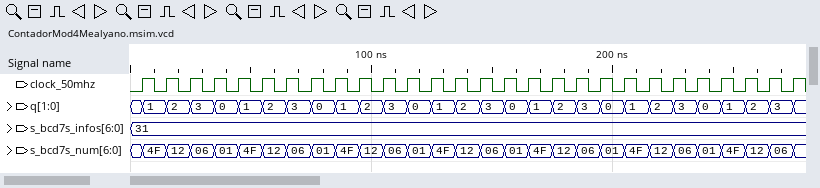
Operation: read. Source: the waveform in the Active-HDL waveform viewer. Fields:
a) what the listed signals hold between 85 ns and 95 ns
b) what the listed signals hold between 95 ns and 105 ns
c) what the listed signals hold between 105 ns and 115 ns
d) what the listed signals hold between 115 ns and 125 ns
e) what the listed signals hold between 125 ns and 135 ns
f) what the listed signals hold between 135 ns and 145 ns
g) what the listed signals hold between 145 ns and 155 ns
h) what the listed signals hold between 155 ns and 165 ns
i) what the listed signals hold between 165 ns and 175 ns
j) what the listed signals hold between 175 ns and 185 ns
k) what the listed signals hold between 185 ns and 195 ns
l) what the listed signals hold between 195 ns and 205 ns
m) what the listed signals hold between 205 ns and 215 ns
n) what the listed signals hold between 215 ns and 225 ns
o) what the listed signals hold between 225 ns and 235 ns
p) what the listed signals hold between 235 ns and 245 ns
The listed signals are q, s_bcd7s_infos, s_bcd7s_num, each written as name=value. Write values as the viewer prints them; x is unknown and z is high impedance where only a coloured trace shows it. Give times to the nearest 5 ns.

q=1, s_bcd7s_infos=31, s_bcd7s_num=4F
q=2, s_bcd7s_infos=31, s_bcd7s_num=12
q=3, s_bcd7s_infos=31, s_bcd7s_num=06
q=0, s_bcd7s_infos=31, s_bcd7s_num=01
q=1, s_bcd7s_infos=31, s_bcd7s_num=4F
q=2, s_bcd7s_infos=31, s_bcd7s_num=12
q=3, s_bcd7s_infos=31, s_bcd7s_num=06
q=0, s_bcd7s_infos=31, s_bcd7s_num=01
q=1, s_bcd7s_infos=31, s_bcd7s_num=4F
q=2, s_bcd7s_infos=31, s_bcd7s_num=12
q=3, s_bcd7s_infos=31, s_bcd7s_num=06
q=0, s_bcd7s_infos=31, s_bcd7s_num=01
q=1, s_bcd7s_infos=31, s_bcd7s_num=4F
q=2, s_bcd7s_infos=31, s_bcd7s_num=12
q=3, s_bcd7s_infos=31, s_bcd7s_num=06
q=0, s_bcd7s_infos=31, s_bcd7s_num=01
